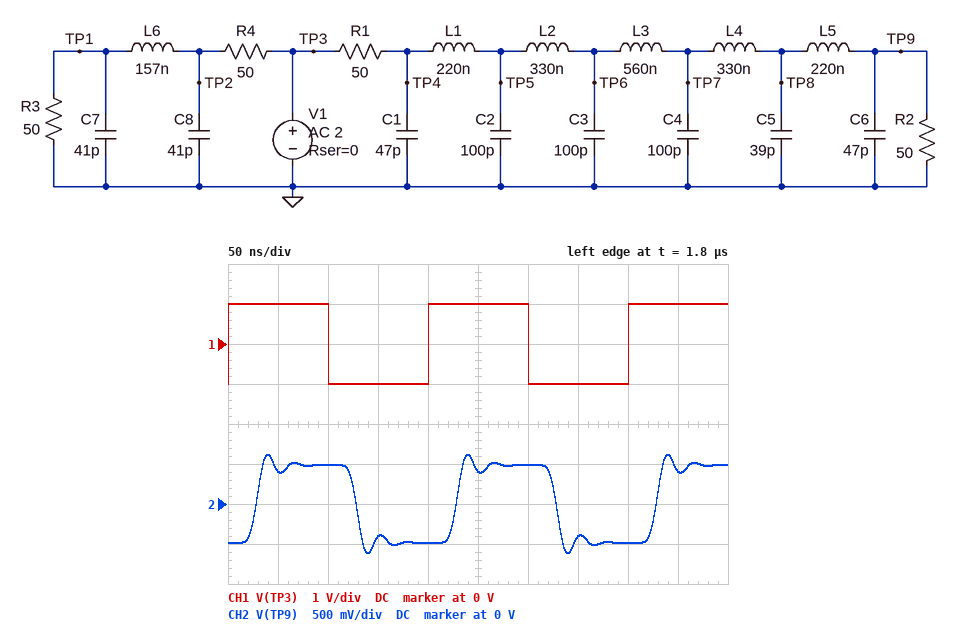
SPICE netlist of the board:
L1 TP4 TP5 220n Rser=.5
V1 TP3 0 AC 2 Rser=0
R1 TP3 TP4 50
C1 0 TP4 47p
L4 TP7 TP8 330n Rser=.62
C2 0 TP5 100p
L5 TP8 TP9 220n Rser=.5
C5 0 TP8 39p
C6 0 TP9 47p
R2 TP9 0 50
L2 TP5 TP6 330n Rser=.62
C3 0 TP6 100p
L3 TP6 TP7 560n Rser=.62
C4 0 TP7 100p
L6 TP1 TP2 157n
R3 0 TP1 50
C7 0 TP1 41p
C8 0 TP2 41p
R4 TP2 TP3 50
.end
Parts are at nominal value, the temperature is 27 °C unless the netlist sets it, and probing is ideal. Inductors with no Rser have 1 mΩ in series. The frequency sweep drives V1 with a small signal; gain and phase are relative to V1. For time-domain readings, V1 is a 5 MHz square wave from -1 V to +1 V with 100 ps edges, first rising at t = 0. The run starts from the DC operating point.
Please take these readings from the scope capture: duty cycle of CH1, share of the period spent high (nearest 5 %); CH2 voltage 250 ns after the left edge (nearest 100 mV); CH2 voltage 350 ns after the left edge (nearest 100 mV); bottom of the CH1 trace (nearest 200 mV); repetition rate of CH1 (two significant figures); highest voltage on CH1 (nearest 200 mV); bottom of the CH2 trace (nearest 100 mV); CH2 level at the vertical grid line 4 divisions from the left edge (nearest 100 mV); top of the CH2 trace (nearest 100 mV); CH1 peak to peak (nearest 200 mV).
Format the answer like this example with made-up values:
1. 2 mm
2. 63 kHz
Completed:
1. 50 %
2. 400 mV
3. -400 mV
4. -1.0 V
5. 5.0 MHz
6. 1.0 V
7. -600 mV
8. -500 mV
9. 600 mV
10. 2.0 V
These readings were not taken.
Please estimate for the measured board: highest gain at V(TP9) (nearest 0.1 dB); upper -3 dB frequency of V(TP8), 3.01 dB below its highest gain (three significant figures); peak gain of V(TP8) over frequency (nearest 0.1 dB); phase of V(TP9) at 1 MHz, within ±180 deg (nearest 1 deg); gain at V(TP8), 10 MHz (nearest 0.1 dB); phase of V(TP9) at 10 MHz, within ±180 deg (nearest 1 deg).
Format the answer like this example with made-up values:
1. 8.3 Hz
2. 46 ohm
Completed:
1. -6.3 dB
2. 41.1 MHz
3. -5.9 dB
4. -10 deg
5. -6.6 dB
6. -97 deg
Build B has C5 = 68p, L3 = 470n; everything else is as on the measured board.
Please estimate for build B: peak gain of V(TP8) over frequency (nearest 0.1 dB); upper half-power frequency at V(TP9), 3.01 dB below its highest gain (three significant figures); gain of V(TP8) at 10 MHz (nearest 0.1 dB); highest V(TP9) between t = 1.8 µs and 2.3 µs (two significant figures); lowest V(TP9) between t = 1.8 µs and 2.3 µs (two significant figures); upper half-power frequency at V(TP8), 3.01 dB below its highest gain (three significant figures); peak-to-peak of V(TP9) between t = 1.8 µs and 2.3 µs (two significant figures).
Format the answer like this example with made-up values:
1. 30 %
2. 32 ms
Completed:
1. -5.6 dB
2. 44.6 MHz
3. -6.4 dB
4. 650 mV
5. -650 mV
6. 47.1 MHz
7. 1.3 V
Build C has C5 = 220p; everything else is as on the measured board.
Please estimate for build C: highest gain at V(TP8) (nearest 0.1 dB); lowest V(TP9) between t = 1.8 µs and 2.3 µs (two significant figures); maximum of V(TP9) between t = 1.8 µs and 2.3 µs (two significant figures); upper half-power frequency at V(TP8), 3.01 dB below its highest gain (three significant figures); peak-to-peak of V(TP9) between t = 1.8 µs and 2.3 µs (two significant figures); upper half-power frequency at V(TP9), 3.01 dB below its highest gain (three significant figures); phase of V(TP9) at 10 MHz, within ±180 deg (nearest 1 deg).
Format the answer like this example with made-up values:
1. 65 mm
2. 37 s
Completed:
1. -5.6 dB
2. -570 mV
3. 570 mV
4. 43.3 MHz
5. 1.1 V
6. 42.7 MHz
7. -117 deg
